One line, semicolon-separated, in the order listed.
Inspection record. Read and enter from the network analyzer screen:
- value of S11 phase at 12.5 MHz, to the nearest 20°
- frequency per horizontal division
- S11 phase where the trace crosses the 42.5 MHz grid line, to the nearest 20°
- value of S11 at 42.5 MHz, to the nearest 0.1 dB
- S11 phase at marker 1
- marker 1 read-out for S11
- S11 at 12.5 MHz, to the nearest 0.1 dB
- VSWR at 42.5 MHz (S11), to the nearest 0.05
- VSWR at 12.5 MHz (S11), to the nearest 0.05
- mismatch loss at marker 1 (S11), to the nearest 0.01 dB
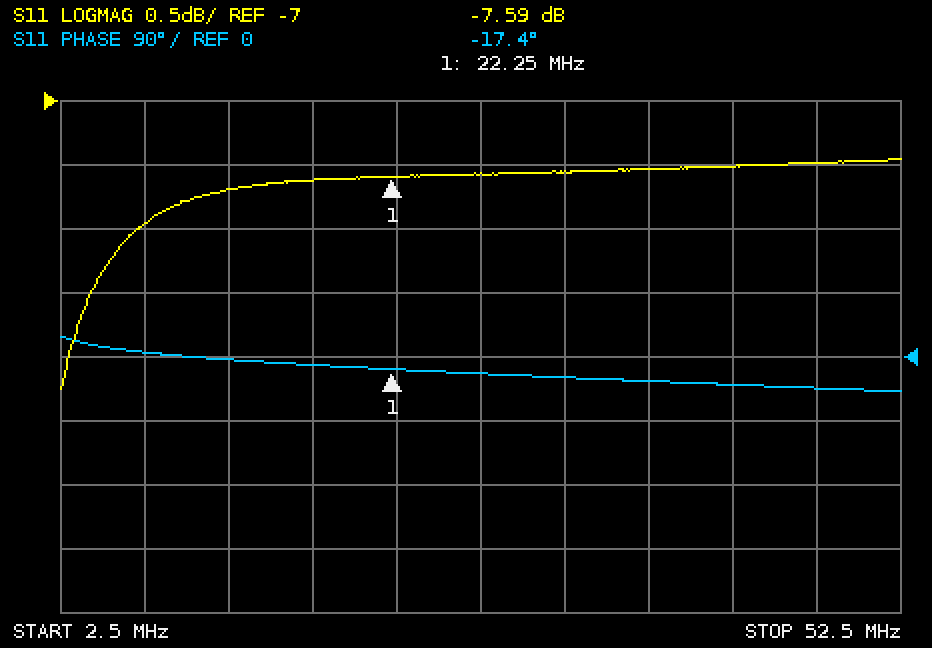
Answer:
0°; 5 MHz; -40°; -7.5 dB; -17.4°; -7.59 dB; -7.7 dB; 2.45; 2.40; 0.83 dB
